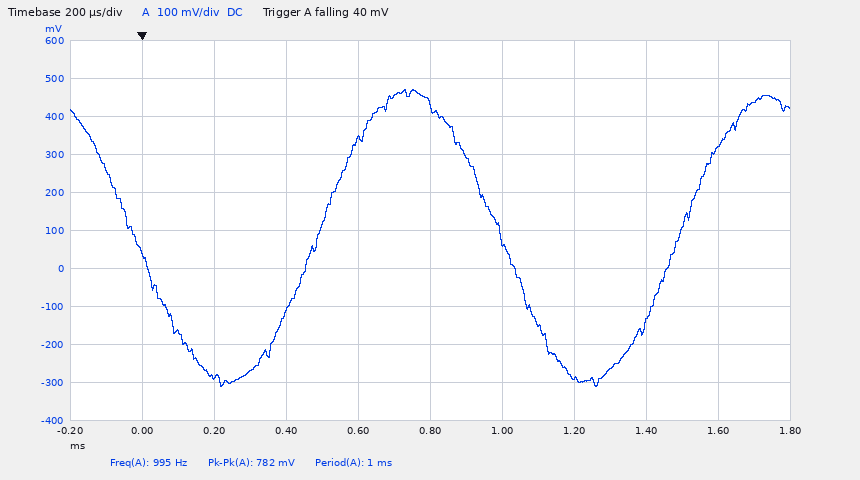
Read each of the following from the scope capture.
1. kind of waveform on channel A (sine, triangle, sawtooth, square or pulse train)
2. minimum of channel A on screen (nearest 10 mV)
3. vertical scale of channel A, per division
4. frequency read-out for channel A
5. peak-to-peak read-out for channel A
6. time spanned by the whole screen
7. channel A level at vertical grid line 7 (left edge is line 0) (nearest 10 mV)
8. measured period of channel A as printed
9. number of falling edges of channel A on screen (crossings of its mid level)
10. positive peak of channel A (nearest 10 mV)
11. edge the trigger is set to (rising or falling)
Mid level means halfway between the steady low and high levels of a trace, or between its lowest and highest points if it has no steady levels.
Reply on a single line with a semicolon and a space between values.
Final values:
sine; -310 mV; 100 mV; 995 Hz; 782 mV; 2 ms; -290 mV; 1 ms; 2; 470 mV; falling
